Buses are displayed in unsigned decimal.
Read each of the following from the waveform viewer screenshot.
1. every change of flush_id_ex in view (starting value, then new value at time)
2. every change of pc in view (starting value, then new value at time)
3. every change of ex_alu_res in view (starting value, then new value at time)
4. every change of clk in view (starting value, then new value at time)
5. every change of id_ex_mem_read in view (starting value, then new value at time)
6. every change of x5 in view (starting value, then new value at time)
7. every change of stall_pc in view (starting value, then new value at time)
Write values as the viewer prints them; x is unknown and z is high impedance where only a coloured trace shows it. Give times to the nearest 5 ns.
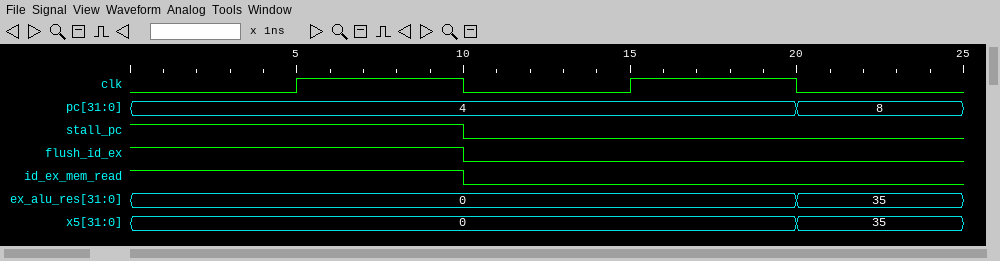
1, 0 at 10 ns
4, 8 at 20 ns
0, 35 at 20 ns
0, 1 at 5 ns, 0 at 10 ns, 1 at 15 ns, 0 at 20 ns
1, 0 at 10 ns
0, 35 at 20 ns
1, 0 at 10 ns
